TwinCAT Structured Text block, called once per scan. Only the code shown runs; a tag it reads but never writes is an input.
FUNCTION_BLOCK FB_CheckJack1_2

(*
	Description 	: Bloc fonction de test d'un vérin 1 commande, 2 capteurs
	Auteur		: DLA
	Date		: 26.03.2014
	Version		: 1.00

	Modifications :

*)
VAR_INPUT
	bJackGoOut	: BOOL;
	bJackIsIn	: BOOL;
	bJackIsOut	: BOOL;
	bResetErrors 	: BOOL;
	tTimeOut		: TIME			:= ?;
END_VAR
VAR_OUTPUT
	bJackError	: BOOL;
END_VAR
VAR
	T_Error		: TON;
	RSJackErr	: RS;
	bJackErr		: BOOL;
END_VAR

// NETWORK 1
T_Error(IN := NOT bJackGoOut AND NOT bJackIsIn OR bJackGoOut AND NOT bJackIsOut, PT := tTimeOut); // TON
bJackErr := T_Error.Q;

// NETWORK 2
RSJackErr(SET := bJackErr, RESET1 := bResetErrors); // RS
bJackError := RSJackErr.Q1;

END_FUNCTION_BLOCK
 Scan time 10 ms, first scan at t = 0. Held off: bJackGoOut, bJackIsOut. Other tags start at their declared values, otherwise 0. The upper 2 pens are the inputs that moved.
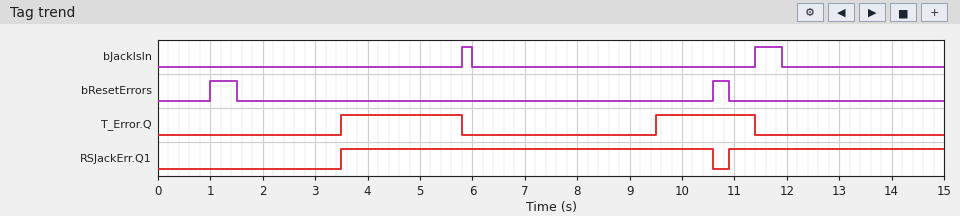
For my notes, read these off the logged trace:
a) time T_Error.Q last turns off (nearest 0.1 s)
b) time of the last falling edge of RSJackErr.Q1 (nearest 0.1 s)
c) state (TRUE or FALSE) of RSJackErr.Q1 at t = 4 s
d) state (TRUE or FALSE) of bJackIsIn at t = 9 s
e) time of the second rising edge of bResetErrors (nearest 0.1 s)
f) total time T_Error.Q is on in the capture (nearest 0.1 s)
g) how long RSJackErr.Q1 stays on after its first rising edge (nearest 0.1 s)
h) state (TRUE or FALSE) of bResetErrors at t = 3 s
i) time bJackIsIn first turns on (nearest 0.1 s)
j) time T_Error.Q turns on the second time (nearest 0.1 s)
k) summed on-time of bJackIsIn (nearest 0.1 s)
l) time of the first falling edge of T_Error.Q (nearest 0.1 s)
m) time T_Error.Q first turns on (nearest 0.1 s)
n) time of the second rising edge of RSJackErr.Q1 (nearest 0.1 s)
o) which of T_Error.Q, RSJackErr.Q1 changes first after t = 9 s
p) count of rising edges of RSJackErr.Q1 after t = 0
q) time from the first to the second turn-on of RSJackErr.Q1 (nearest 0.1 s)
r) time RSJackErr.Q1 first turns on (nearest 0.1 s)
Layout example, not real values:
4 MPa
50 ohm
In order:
11.4 s
10.6 s
TRUE
FALSE
10.6 s
4.2 s
7.1 s
FALSE
5.8 s
9.5 s
0.7 s
5.8 s
3.5 s
10.9 s
T_Error.Q
2
7.4 s
3.5 s
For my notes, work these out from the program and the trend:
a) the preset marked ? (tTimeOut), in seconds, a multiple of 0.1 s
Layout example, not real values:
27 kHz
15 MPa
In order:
3.5 s
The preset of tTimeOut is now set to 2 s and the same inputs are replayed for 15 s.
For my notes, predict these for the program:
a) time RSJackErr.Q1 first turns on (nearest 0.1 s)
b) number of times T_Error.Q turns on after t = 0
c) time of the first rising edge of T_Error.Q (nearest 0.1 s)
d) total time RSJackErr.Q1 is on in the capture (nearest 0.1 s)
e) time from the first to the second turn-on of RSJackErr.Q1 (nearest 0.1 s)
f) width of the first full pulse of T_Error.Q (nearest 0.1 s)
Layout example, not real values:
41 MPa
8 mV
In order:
2.0 s
3
2.0 s
12.7 s
8.9 s
3.8 s
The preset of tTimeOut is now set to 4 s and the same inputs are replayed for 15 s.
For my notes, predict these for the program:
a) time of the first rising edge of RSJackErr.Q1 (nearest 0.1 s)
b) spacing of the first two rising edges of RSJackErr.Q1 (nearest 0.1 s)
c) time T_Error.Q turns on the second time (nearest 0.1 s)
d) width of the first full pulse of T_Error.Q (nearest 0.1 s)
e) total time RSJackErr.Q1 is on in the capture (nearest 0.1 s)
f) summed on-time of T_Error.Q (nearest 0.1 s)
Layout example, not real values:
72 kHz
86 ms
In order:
4.0 s
6.9 s
10.0 s
1.8 s
10.7 s
3.2 s
